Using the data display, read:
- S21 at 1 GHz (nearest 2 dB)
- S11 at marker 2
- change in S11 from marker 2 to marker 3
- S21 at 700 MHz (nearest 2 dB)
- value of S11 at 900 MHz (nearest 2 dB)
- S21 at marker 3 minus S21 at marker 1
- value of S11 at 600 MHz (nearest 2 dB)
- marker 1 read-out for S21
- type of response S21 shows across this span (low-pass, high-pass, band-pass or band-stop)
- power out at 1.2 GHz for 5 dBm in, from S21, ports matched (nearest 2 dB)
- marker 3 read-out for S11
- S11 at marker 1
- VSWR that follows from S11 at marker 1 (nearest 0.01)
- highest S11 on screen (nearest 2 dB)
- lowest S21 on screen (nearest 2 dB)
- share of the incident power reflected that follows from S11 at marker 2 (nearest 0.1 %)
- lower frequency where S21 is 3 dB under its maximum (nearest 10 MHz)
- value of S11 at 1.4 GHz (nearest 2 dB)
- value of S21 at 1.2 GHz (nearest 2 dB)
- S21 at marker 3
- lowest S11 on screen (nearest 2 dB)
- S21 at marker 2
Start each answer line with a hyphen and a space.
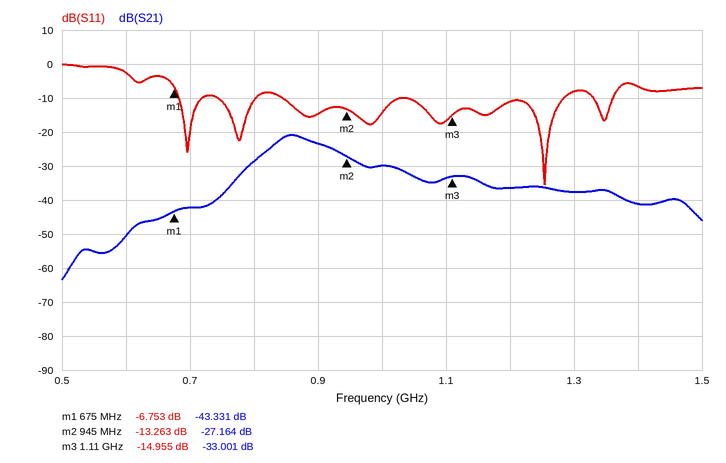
- -30 dB
- -13.263 dB
- -1.692 dB
- -42 dB
- -14 dB
- 10.330 dB
- -2 dB
- -43.331 dB
- band-pass
- -32 dBm
- -14.955 dB
- -6.753 dB
- 2.70
- 0 dB
- -64 dB
- 4.7 %
- 830 MHz
- -6 dB
- -36 dB
- -33.001 dB
- -36 dB
- -27.164 dB
